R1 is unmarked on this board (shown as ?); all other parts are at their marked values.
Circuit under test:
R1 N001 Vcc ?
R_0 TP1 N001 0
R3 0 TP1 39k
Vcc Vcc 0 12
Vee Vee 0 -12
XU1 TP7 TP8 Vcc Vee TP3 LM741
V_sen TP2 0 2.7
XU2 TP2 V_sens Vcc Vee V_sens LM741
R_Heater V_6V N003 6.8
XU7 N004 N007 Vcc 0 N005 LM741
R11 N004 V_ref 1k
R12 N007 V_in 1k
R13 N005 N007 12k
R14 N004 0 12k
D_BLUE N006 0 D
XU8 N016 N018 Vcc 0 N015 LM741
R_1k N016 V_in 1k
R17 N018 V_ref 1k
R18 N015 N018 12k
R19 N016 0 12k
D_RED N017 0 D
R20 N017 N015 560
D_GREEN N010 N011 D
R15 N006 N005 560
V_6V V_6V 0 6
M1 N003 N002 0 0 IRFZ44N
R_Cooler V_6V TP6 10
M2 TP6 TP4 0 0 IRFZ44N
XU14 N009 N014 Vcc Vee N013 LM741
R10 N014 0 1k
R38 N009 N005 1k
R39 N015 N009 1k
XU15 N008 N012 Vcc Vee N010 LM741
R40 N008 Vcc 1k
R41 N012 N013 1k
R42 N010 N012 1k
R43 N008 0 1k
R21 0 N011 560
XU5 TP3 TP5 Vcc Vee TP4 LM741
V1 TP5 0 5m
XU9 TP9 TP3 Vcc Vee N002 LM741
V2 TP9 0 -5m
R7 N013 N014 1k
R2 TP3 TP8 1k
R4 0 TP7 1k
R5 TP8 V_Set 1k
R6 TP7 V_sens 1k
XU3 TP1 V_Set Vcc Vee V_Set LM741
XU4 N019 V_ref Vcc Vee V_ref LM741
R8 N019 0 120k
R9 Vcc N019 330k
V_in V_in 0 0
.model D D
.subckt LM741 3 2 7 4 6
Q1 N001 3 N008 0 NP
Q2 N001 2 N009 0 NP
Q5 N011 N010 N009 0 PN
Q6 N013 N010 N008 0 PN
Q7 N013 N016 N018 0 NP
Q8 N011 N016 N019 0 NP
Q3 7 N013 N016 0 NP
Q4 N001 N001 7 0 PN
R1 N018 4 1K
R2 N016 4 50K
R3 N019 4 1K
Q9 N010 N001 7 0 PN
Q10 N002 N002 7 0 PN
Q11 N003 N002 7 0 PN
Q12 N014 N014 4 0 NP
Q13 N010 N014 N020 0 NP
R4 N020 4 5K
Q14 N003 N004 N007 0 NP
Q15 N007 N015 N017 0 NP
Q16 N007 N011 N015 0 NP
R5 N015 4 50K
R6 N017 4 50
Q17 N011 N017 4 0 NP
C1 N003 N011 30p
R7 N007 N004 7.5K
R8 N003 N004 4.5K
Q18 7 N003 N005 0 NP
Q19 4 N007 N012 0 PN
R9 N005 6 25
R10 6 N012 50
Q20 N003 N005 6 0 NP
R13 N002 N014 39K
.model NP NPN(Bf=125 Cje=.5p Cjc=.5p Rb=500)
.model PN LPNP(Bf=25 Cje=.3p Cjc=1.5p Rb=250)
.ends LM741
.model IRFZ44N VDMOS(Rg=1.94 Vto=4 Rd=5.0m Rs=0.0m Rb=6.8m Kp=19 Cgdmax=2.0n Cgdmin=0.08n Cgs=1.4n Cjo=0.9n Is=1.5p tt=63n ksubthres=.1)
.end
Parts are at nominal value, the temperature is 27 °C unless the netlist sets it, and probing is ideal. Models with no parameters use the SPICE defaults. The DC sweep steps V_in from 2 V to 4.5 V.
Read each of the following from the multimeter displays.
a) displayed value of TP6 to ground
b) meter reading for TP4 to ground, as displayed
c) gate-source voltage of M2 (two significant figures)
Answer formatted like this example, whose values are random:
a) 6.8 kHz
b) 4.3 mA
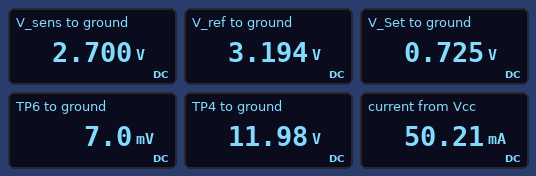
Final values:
a) 7.0 mV
b) 11.98 V
c) 12 V
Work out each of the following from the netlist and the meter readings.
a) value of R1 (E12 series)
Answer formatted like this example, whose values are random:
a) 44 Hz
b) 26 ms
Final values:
a) 220 kΩ
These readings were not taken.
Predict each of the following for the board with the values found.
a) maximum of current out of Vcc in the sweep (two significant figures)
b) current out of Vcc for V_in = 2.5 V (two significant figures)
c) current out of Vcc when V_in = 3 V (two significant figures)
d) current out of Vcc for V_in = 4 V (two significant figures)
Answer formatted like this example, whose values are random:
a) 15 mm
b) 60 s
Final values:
a) 50 mA
b) 44 mA
c) 38 mA
d) 48 mA
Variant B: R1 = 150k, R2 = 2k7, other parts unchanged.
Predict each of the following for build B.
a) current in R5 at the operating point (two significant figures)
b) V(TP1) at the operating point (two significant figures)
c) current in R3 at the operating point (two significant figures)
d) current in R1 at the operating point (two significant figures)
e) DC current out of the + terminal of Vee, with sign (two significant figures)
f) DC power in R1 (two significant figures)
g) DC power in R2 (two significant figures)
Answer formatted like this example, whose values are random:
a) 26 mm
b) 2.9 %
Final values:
a) 290 µA
b) 1.1 V
c) 27 µA
d) 73 µA
e) -12 mA
f) 800 µW
g) 220 µW
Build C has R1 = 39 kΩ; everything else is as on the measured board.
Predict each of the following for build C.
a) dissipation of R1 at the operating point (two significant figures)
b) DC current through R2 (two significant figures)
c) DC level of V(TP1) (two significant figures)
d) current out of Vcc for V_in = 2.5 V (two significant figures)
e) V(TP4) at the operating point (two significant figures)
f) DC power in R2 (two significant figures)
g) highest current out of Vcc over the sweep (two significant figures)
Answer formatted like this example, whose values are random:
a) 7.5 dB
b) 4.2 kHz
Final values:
a) 1.6 mW
b) 2.7 mA
c) 4.1 V
d) 47 mA
e) -11 V
f) 7.5 mW
g) 52 mA
